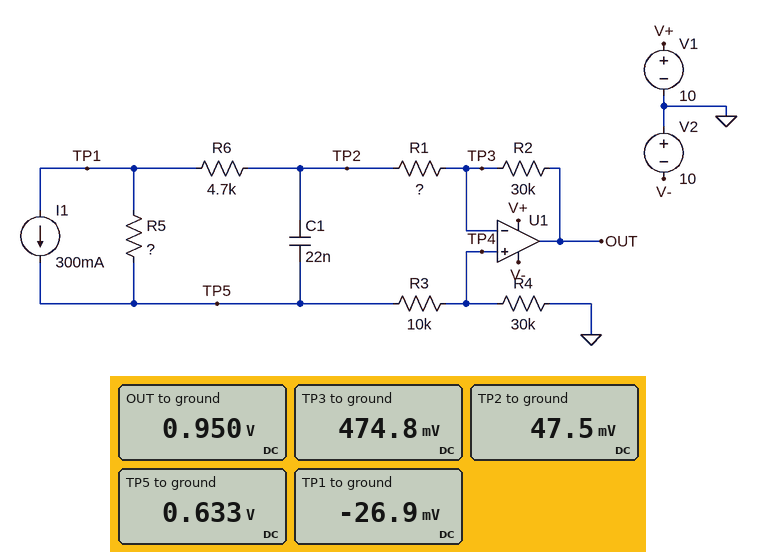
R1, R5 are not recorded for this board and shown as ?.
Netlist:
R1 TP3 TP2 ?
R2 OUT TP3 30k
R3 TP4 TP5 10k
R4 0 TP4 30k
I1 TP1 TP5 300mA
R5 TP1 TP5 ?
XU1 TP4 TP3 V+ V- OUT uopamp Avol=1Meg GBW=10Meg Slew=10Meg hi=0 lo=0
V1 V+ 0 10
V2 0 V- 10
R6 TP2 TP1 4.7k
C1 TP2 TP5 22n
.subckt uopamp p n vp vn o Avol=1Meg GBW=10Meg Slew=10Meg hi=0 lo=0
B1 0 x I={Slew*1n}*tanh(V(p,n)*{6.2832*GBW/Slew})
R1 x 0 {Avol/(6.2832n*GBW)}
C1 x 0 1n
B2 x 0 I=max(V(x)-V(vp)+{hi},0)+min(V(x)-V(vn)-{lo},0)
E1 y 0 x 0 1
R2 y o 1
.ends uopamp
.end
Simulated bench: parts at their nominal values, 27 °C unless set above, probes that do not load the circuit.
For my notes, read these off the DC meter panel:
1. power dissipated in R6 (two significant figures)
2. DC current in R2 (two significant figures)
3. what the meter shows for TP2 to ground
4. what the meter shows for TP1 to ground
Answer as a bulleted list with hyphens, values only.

- 1.2 µW
- 16 µA
- 47.5 mV
- -26.9 mV
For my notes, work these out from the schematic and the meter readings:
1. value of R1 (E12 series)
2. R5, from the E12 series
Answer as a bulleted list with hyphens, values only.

- 27 kΩ
- 2.2 Ω
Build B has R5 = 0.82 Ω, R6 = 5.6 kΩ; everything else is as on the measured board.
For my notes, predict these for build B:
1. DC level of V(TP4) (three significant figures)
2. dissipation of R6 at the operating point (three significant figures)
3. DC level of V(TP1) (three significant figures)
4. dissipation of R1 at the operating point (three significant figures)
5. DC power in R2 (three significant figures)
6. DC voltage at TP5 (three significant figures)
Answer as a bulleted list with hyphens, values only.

- 173 mV
- 187 nW
- -15.0 mV
- 900 nW
- 1.00 µW
- 231 mV
